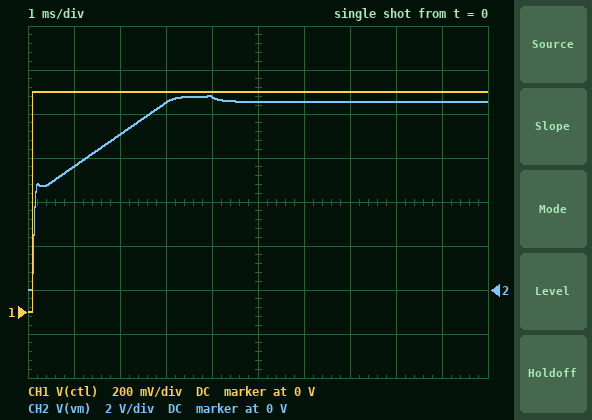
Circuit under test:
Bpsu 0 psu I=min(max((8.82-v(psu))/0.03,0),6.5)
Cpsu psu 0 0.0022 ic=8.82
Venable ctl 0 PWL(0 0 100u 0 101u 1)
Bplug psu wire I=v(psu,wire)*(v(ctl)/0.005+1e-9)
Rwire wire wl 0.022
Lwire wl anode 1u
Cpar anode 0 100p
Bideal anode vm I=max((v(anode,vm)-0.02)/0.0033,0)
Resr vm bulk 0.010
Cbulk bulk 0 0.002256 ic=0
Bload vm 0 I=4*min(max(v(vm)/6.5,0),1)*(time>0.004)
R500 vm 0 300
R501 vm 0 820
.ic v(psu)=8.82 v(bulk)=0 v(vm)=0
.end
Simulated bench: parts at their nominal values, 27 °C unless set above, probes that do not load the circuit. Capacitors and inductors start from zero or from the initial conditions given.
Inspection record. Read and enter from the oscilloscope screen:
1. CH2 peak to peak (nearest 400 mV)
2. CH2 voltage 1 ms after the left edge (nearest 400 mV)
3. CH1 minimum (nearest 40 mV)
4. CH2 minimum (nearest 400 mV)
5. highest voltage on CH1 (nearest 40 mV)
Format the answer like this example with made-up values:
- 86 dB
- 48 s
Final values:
- 8.8 V
- 5.6 V
- 0 V
- 0 V
- 1.00 V
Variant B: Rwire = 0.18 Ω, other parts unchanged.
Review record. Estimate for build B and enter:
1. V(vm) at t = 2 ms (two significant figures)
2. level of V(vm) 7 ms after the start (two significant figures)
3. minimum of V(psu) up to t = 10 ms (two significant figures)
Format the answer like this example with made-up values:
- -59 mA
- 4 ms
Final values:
- 6.8 V
- 7.9 V
- 5.8 V
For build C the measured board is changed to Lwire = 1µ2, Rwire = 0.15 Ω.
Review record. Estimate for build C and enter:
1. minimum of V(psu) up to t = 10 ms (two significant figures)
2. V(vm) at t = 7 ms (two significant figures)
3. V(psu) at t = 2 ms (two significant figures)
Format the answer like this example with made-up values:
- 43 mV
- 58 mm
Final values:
- 5.6 V
- 8.0 V
- 7.4 V
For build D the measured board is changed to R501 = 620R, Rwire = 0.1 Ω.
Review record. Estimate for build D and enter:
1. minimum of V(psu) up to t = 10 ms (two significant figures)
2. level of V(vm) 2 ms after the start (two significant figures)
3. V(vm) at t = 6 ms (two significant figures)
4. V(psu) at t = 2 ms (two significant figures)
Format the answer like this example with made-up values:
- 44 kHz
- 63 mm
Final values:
- 5.3 V
- 6.9 V
- 8.2 V
- 7.3 V
